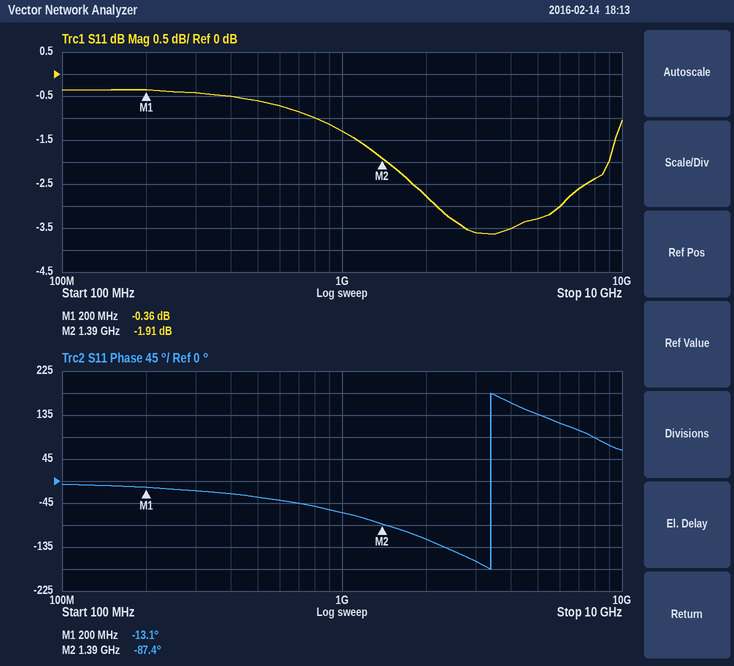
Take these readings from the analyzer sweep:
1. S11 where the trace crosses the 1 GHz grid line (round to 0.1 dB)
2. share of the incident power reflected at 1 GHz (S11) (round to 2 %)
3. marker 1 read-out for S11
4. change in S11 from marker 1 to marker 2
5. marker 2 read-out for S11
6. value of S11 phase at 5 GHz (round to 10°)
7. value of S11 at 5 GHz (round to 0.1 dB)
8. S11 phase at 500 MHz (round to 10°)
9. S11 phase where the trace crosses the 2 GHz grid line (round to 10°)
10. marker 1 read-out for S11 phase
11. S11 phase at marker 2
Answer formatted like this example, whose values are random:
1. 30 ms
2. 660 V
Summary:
1. -1.3 dB
2. 74 %
3. -0.36 dB
4. -1.55 dB
5. -1.91 dB
6. 140°
7. -3.3 dB
8. -30°
9. -120°
10. -13.1°
11. -87.4°
